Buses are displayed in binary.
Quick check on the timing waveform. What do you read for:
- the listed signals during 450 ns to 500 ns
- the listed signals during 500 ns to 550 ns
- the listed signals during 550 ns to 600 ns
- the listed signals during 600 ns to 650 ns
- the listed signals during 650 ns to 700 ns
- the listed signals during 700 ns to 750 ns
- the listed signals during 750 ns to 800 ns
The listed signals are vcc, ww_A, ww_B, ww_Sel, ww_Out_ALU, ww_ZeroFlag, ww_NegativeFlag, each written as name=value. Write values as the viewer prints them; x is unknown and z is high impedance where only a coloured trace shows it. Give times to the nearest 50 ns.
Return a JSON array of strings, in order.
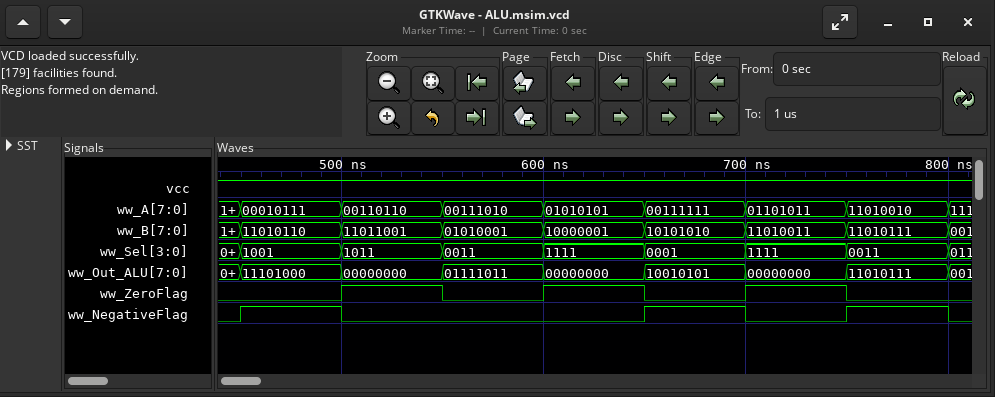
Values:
["vcc=1, ww_A=00010111, ww_B=11010110, ww_Sel=1001, ww_Out_ALU=11101000, ww_ZeroFlag=0, ww_NegativeFlag=1", "vcc=1, ww_A=00110110, ww_B=11011001, ww_Sel=1011, ww_Out_ALU=00000000, ww_ZeroFlag=1, ww_NegativeFlag=0", "vcc=1, ww_A=00111010, ww_B=01010001, ww_Sel=0011, ww_Out_ALU=01111011, ww_ZeroFlag=0, ww_NegativeFlag=0", "vcc=1, ww_A=01010101, ww_B=10000001, ww_Sel=1111, ww_Out_ALU=00000000, ww_ZeroFlag=1, ww_NegativeFlag=0", "vcc=1, ww_A=00111111, ww_B=10101010, ww_Sel=0001, ww_Out_ALU=10010101, ww_ZeroFlag=0, ww_NegativeFlag=1", "vcc=1, ww_A=01101011, ww_B=11010011, ww_Sel=1111, ww_Out_ALU=00000000, ww_ZeroFlag=1, ww_NegativeFlag=0", "vcc=1, ww_A=11010010, ww_B=11010111, ww_Sel=0011, ww_Out_ALU=11010111, ww_ZeroFlag=0, ww_NegativeFlag=1"]
